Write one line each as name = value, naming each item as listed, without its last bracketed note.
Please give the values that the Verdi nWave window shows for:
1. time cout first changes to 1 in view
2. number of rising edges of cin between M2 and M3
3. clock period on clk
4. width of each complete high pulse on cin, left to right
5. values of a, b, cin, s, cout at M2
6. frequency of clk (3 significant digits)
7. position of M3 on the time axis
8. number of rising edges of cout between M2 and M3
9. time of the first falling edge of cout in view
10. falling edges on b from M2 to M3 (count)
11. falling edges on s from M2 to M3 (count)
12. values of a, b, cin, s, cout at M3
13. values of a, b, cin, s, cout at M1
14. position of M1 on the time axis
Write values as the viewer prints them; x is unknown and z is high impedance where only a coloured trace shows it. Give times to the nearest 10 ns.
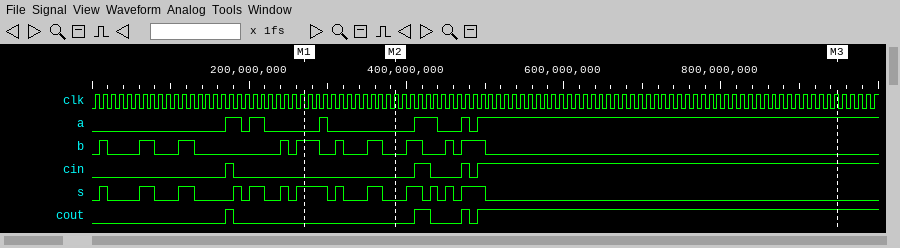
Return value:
time cout first changes to 1 in view = 170 ns
number of rising edges of cin between M2 and M3 = 3
clock period on clk = 10 ns
width of each complete high pulse on cin, left to right = 10 ns, 20 ns, 10 ns
values of a, b, cin, s, cout at M2 = a=0, b=0, cin=0, s=0, cout=0
frequency of clk = 100 MHz
position of M3 on the time axis = 950 ns
number of rising edges of cout between M2 and M3 = 3
time of the first falling edge of cout in view = 180 ns
falling edges on b from M2 to M3 = 3
falling edges on s from M2 to M3 = 4
values of a, b, cin, s, cout at M3 = a=1, b=0, cin=1, s=0, cout=1
values of a, b, cin, s, cout at M1 = a=0, b=1, cin=0, s=1, cout=0
position of M1 on the time axis = 270 ns
